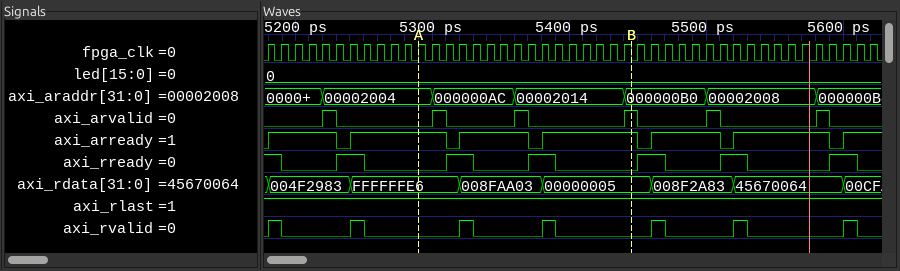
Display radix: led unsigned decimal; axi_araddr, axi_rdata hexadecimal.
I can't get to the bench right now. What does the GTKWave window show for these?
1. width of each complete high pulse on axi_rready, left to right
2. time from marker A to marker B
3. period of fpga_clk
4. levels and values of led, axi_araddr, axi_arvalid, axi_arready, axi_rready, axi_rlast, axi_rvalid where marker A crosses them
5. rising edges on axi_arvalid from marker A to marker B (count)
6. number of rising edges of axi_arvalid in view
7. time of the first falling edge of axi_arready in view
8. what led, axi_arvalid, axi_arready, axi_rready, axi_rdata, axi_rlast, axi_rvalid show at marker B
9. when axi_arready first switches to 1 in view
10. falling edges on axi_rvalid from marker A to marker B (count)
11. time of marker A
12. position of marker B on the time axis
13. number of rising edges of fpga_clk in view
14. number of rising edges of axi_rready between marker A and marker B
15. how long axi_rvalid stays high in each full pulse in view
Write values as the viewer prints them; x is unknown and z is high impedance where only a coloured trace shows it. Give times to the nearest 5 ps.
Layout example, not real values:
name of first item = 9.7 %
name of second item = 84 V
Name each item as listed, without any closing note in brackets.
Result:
width of each complete high pulse on axi_rready, left to right = 20 ps, 20 ps, 20 ps, 20 ps, 20 ps, 20 ps
time from marker A to marker B = 155 ps
period of fpga_clk = 10 ps
levels and values of led, axi_araddr, axi_arvalid, axi_arready, axi_rready, axi_rlast, axi_rvalid where marker A crosses them = led=0, axi_araddr=00002004, axi_arvalid=0, axi_arready=1, axi_rready=0, axi_rlast=1, axi_rvalid=0
rising edges on axi_arvalid from marker A to marker B = 3
number of rising edges of axi_arvalid in view = 6
time of the first falling edge of axi_arready in view = 5230 ps
what led, axi_arvalid, axi_arready, axi_rready, axi_rdata, axi_rlast, axi_rvalid show at marker B = led=0, axi_arvalid=1, axi_arready=1, axi_rready=0, axi_rdata=00000005, axi_rlast=1, axi_rvalid=0
when axi_arready first switches to 1 in view = 5180 ps
falling edges on axi_rvalid from marker A to marker B = 2
time of marker A = 5290 ps
position of marker B on the time axis = 5445 ps
number of rising edges of fpga_clk in view = 45
number of rising edges of axi_rready between marker A and marker B = 2
how long axi_rvalid stays high in each full pulse in view = 10 ps, 10 ps, 10 ps, 10 ps, 10 ps, 10 ps, 10 ps
